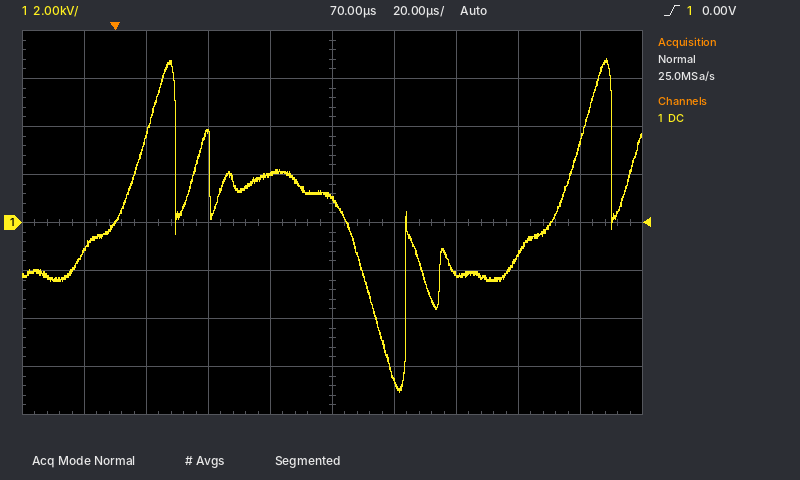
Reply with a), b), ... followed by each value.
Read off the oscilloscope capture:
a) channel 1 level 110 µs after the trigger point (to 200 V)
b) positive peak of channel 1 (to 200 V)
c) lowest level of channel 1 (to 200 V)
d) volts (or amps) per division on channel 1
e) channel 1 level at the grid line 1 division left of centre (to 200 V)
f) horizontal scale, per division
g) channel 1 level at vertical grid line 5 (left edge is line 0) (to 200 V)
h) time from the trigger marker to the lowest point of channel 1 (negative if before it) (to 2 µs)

a) -2.2 kV
b) 6.8 kV
c) -7.0 kV
d) 2 kV
e) 2.0 kV
f) 20 µs
g) 1.0 kV
h) +92 µs
